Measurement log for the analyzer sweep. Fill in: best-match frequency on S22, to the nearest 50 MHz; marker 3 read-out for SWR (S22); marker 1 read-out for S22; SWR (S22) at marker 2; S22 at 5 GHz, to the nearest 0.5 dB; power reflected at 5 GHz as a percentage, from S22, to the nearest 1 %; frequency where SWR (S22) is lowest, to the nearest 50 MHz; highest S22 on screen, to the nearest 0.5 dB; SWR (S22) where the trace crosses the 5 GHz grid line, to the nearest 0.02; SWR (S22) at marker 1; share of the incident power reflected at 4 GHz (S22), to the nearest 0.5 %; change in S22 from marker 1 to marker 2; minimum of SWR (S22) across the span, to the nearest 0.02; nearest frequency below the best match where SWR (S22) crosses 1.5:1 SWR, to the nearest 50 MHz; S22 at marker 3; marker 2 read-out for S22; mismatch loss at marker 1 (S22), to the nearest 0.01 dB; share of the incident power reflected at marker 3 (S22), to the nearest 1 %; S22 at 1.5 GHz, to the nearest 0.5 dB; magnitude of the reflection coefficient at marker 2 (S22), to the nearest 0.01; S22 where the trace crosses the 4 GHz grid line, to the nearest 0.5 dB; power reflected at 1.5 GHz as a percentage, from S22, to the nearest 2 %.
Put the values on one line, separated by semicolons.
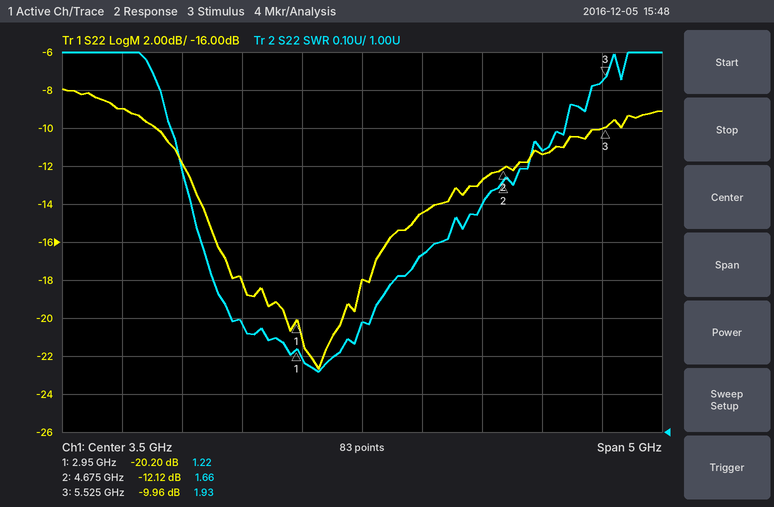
3.15 GHz; 1.93; -20.20 dB; 1.66; -11.5 dB; 7 %; 3.15 GHz; -8.0 dB; 1.74; 1.22; 3.5 %; 8.08 dB; 1.16; 2.15 GHz; -9.96 dB; -12.12 dB; 0.04 dB; 10 %; -9.0 dB; 0.25; -14.5 dB; 12 %
